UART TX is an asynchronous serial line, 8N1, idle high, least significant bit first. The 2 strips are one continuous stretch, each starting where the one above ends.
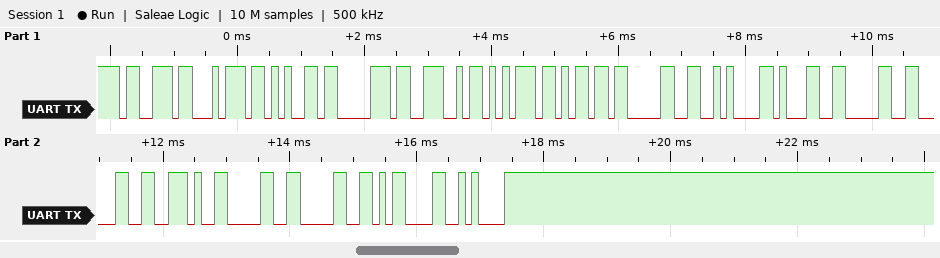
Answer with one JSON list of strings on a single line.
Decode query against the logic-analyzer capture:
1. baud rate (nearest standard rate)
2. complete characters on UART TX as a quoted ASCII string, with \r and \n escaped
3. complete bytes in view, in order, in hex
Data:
["9600 baud", "\"stepNum0\\n100.00\\r\\n\"", "73 74 65 70 4E 75 6D 30 0A 31 30 30 2E 30 30 0D 0A"]
